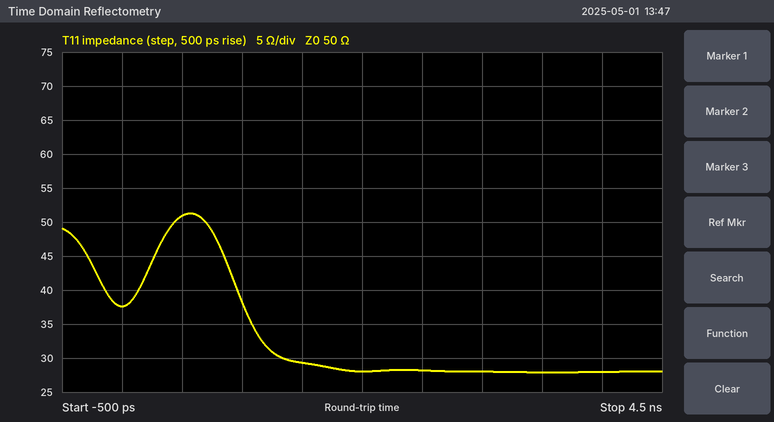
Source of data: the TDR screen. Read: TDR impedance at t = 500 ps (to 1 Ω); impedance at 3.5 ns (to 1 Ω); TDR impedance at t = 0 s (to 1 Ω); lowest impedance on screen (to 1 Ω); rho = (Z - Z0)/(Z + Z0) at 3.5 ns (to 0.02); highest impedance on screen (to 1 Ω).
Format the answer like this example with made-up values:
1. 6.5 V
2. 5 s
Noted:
1. 51 Ω
2. 28 Ω
3. 38 Ω
4. 28 Ω
5. -0.28
6. 51 Ω
